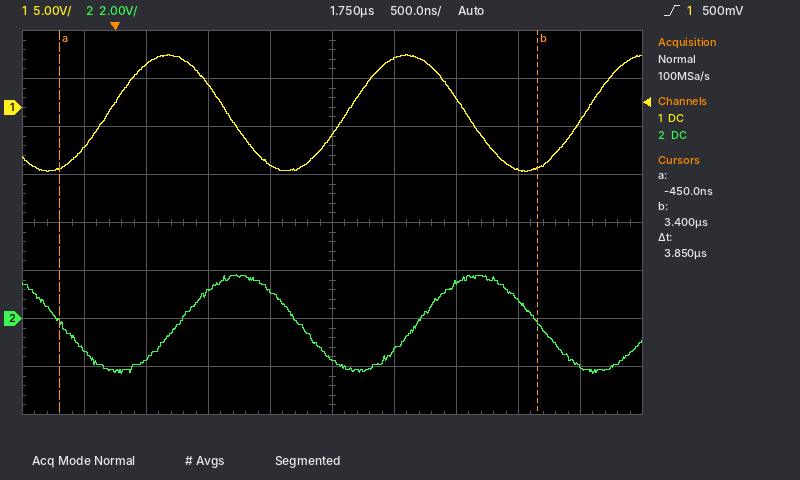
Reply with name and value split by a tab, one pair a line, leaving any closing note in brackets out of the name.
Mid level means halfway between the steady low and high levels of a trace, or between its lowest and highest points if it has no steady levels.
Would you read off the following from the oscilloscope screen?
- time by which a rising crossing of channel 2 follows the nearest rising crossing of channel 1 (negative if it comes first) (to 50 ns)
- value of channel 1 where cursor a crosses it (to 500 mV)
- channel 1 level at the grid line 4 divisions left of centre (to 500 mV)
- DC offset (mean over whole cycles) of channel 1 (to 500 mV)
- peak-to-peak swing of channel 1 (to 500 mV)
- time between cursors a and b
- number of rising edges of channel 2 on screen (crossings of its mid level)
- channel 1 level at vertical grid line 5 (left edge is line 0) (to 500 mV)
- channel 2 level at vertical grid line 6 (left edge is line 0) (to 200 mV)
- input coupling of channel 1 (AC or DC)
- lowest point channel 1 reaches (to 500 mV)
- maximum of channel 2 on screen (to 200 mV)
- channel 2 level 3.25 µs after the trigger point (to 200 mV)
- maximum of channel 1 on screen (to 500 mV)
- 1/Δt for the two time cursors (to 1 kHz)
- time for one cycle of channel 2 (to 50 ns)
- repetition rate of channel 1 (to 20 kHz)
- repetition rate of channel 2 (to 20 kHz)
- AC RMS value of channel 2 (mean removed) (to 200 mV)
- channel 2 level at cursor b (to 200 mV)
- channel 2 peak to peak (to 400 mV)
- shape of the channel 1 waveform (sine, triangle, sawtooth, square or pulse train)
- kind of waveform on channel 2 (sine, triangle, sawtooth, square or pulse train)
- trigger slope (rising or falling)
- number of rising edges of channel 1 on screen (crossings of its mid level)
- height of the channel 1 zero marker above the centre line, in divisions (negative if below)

time by which a rising crossing of channel 2 follows the nearest rising crossing of channel 1 (negative if it comes first)	+550 ns
value of channel 1 where cursor a crosses it	-6.5 V
channel 1 level at the grid line 4 divisions left of centre	-4.0 V
DC offset (mean over whole cycles) of channel 1	-500 mV
peak-to-peak swing of channel 1	12.0 V
time between cursors a and b	3.85 µs
number of rising edges of channel 2 on screen	2
channel 1 level at vertical grid line 5 (left edge is line 0)	-3.0 V
channel 2 level at vertical grid line 6 (left edge is line 0)	-1.4 V
input coupling of channel 1	DC
lowest point channel 1 reaches	-6.5 V
maximum of channel 2 on screen	1.8 V
channel 2 level 3.25 µs after the trigger point	800 mV
maximum of channel 1 on screen	5.5 V
1/Δt for the two time cursors	260 kHz
time for one cycle of channel 2	1.90 µs
repetition rate of channel 1	520 kHz
repetition rate of channel 2	520 kHz
AC RMS value of channel 2 (mean removed)	1.4 V
channel 2 level at cursor b	-200 mV
channel 2 peak to peak	4.0 V
shape of the channel 1 waveform	sine
kind of waveform on channel 2	sine
trigger slope	rising
number of rising edges of channel 1 on screen	3
height of the channel 1 zero marker above the centre line, in divisions	+2.4 div
